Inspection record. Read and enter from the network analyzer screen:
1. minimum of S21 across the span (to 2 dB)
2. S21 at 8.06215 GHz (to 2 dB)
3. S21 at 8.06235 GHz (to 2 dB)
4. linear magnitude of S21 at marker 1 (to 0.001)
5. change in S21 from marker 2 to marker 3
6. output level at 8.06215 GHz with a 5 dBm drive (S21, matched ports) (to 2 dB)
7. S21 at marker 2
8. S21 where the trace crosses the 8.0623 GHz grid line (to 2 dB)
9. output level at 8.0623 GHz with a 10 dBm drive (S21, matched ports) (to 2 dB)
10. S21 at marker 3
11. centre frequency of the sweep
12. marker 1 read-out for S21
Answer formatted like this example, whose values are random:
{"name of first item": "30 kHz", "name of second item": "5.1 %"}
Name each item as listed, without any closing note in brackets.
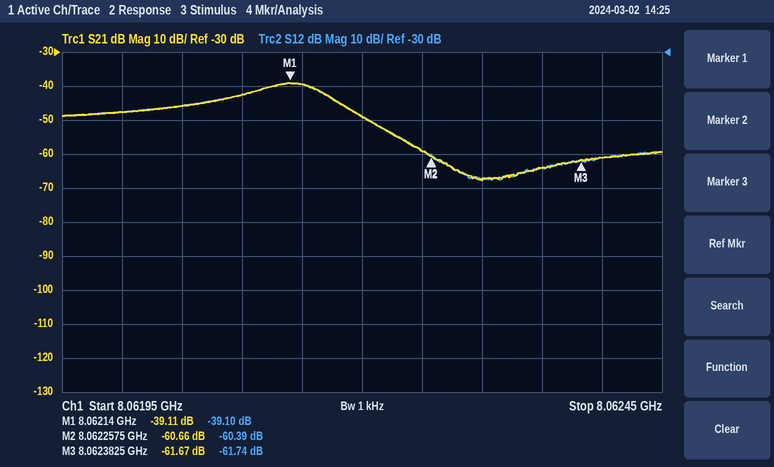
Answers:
{"minimum of S21 across the span": "-68 dB", "S21 at 8.06215 GHz": "-40 dB", "S21 at 8.06235 GHz": "-64 dB", "linear magnitude of S21 at marker 1": "0.011", "change in S21 from marker 2 to marker 3": "-1.01 dB", "output level at 8.06215 GHz with a 5 dBm drive (S21, matched ports)": "-34 dBm", "S21 at marker 2": "-60.66 dB", "S21 where the trace crosses the 8.0623 GHz grid line": "-68 dB", "output level at 8.0623 GHz with a 10 dBm drive (S21, matched ports)": "-58 dBm", "S21 at marker 3": "-61.67 dB", "centre frequency of the sweep": "8.0622 GHz", "marker 1 read-out for S21": "-39.11 dB"}
